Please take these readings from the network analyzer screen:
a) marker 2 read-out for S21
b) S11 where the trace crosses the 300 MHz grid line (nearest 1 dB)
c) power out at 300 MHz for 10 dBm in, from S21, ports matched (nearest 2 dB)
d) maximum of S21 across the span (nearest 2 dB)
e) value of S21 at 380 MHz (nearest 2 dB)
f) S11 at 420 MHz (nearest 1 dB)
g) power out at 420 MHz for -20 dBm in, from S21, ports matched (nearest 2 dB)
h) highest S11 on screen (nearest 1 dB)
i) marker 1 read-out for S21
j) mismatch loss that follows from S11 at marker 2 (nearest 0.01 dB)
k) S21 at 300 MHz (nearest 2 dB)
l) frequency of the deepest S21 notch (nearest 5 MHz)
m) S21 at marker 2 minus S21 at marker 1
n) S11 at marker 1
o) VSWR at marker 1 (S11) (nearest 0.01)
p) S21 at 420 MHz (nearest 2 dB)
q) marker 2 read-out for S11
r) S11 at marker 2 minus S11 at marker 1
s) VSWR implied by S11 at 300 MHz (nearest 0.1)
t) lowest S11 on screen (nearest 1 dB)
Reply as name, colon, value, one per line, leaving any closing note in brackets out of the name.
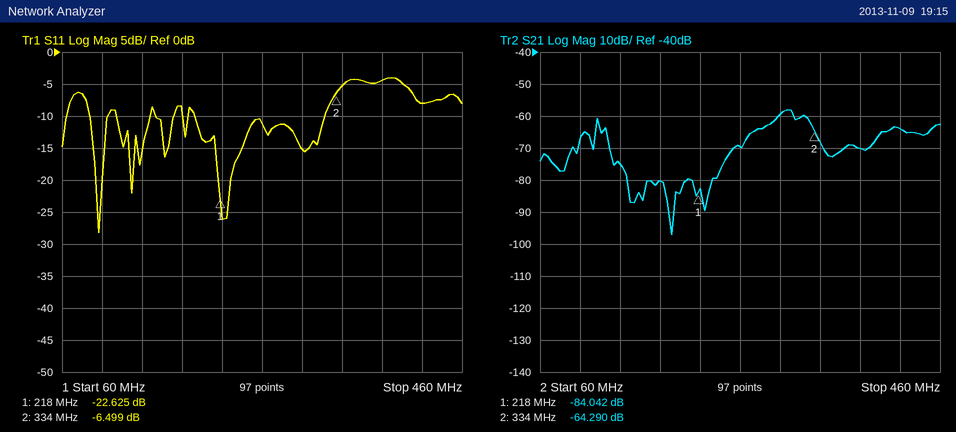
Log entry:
marker 2 read-out for S21: -64.290 dB
S11 where the trace crosses the 300 MHz grid line: -15 dB
power out at 300 MHz for 10 dBm in, from S21, ports matched: -50 dBm
maximum of S21 across the span: -58 dB
value of S21 at 380 MHz: -70 dB
S11 at 420 MHz: -8 dB
power out at 420 MHz for -20 dBm in, from S21, ports matched: -84 dBm
highest S11 on screen: -4 dB
marker 1 read-out for S21: -84.042 dB
mismatch loss that follows from S11 at marker 2: 1.10 dB
S21 at 300 MHz: -60 dB
frequency of the deepest S21 notch: 190 MHz
S21 at marker 2 minus S21 at marker 1: 19.752 dB
S11 at marker 1: -22.625 dB
VSWR at marker 1 (S11): 1.16
S21 at 420 MHz: -64 dB
marker 2 read-out for S11: -6.499 dB
S11 at marker 2 minus S11 at marker 1: 16.126 dB
VSWR implied by S11 at 300 MHz: 1.4
lowest S11 on screen: -28 dB
